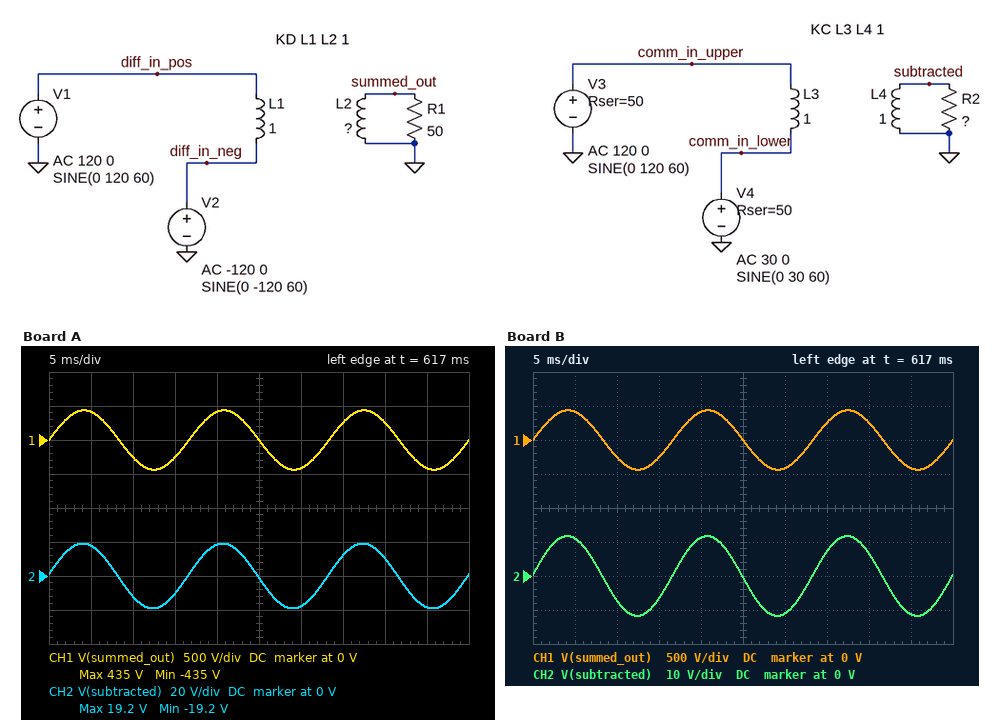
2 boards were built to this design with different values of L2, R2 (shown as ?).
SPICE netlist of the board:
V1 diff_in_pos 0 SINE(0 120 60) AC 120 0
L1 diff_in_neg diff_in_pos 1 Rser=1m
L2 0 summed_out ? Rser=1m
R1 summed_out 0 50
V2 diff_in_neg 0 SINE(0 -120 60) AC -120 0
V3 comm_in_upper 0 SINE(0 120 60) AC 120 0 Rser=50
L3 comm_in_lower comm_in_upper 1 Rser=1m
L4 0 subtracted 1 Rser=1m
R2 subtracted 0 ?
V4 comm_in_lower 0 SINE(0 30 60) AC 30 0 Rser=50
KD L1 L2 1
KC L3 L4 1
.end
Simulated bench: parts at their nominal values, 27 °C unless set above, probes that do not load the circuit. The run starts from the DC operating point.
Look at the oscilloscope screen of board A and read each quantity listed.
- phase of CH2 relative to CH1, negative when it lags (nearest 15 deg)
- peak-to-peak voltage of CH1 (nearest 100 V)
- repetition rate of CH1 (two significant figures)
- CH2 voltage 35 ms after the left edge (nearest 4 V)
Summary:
0 deg
900 V
60 Hz
12 V
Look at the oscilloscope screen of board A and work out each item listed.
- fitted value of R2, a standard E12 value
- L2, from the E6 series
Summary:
27 Ω
3.3 H
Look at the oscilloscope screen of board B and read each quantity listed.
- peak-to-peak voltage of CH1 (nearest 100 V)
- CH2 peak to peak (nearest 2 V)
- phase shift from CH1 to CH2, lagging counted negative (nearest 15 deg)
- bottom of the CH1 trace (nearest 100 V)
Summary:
900 V
24 V
0 deg
-400 V
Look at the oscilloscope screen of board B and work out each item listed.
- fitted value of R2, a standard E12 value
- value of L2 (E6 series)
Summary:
15 Ω
3.3 H
